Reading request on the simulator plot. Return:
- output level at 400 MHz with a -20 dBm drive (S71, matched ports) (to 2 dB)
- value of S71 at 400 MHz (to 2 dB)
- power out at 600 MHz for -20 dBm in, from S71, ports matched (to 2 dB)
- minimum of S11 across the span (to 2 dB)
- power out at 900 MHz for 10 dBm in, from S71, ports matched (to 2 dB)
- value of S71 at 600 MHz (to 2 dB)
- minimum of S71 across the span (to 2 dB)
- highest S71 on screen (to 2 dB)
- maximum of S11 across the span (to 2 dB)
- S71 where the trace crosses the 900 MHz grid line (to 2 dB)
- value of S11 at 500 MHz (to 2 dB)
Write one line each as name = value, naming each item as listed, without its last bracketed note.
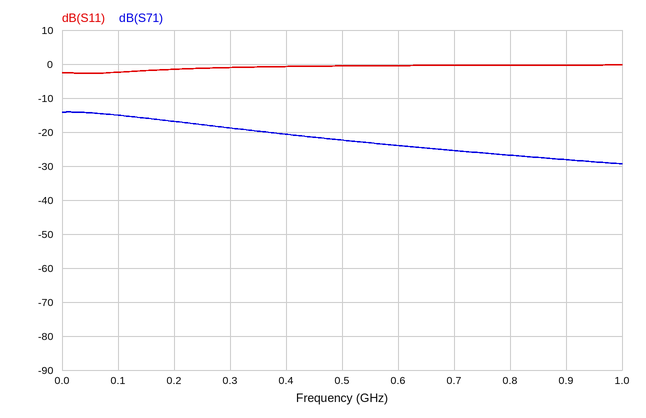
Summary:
output level at 400 MHz with a -20 dBm drive (S71, matched ports) = -40 dBm
value of S71 at 400 MHz = -20 dB
power out at 600 MHz for -20 dBm in, from S71, ports matched = -44 dBm
minimum of S11 across the span = -2 dB
power out at 900 MHz for 10 dBm in, from S71, ports matched = -18 dBm
value of S71 at 600 MHz = -24 dB
minimum of S71 across the span = -30 dB
highest S71 on screen = -14 dB
maximum of S11 across the span = 0 dB
S71 where the trace crosses the 900 MHz grid line = -28 dB
value of S11 at 500 MHz = 0 dB
